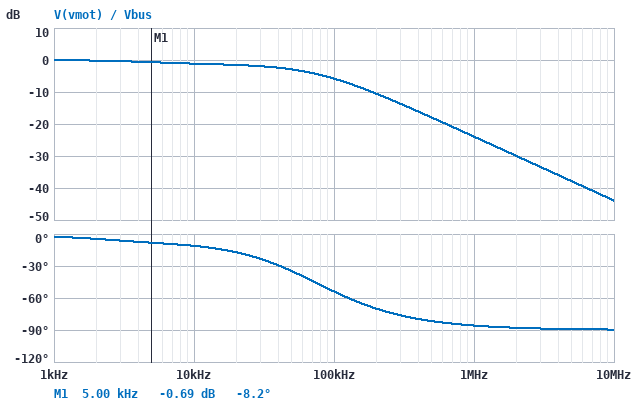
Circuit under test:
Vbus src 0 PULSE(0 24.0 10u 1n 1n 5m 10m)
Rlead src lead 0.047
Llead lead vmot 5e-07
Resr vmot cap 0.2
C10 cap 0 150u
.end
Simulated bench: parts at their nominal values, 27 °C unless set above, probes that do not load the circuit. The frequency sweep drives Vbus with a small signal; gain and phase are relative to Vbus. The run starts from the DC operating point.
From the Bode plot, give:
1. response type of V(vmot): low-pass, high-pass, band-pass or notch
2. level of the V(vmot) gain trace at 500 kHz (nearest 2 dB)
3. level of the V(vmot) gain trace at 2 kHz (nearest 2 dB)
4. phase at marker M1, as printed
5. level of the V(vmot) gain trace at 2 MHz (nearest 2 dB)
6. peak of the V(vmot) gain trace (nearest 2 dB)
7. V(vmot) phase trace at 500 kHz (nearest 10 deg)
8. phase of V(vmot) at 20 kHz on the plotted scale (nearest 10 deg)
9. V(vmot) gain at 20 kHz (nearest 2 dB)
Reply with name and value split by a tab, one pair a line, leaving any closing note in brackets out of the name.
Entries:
response type of V(vmot): low-pass, high-pass, band-pass or notch	low-pass
level of the V(vmot) gain trace at 500 kHz	-18 dB
level of the V(vmot) gain trace at 2 kHz	0 dB
phase at marker M1, as printed	-8.2 deg
level of the V(vmot) gain trace at 2 MHz	-30 dB
peak of the V(vmot) gain trace	0 dB
V(vmot) phase trace at 500 kHz	-80 deg
phase of V(vmot) at 20 kHz on the plotted scale	-20 deg
V(vmot) gain at 20 kHz	-2 dB
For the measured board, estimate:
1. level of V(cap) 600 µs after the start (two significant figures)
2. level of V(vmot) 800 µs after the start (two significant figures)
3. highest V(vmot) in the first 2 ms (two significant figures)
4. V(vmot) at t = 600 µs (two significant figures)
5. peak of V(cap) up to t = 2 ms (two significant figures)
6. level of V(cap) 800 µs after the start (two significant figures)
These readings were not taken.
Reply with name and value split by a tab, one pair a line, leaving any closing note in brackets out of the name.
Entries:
level of V(cap) 600 µs after the start	24 V
level of V(vmot) 800 µs after the start	24 V
highest V(vmot) in the first 2 ms	24 V
V(vmot) at t = 600 µs	24 V
peak of V(cap) up to t = 2 ms	24 V
level of V(cap) 800 µs after the start	24 V
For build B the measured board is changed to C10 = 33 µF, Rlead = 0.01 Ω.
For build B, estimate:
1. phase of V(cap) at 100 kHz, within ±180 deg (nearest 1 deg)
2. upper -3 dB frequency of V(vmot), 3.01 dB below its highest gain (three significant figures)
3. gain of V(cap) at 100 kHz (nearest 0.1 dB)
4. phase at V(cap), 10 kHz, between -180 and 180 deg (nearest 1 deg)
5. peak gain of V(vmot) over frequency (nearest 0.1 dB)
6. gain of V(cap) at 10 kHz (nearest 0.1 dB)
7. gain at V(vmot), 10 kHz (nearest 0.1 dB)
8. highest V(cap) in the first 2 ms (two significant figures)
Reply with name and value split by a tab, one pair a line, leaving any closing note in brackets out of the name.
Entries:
phase of V(cap) at 100 kHz, within ±180 deg	-142 deg
upper -3 dB frequency of V(vmot), 3.01 dB below its highest gain	69.2 kHz
gain of V(cap) at 100 kHz	-16.9 dB
phase at V(cap), 10 kHz, between -180 and 180 deg	-25 deg
peak gain of V(vmot) over frequency	1.3 dB
gain of V(cap) at 10 kHz	-0.3 dB
gain at V(vmot), 10 kHz	0.4 dB
highest V(cap) in the first 2 ms	24 V
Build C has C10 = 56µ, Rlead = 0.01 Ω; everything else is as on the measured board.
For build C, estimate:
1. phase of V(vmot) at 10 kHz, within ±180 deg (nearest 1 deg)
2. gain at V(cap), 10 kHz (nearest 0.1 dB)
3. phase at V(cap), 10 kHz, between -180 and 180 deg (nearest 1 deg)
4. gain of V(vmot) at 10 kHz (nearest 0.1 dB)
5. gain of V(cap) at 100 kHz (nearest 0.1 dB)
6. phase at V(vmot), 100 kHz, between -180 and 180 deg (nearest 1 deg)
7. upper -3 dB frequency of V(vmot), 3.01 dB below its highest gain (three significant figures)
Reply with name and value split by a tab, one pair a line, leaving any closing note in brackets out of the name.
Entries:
phase of V(vmot) at 10 kHz, within ±180 deg	-5 deg
gain at V(cap), 10 kHz	-1.3 dB
phase at V(cap), 10 kHz, between -180 and 180 deg	-40 deg
gain of V(vmot) at 10 kHz	0.5 dB
gain of V(cap) at 100 kHz	-21.9 dB
phase at V(vmot), 100 kHz, between -180 and 180 deg	-62 deg
upper -3 dB frequency of V(vmot), 3.01 dB below its highest gain	65.2 kHz
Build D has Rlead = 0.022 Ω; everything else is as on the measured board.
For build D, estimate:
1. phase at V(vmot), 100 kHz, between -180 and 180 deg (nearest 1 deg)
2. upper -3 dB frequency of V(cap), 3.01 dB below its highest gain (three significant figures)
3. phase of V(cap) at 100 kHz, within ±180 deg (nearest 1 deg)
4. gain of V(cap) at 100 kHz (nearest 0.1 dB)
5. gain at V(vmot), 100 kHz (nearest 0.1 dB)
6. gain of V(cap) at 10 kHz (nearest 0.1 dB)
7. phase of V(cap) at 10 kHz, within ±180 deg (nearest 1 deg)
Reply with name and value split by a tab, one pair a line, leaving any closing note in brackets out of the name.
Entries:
phase at V(vmot), 100 kHz, between -180 and 180 deg	-57 deg
upper -3 dB frequency of V(cap), 3.01 dB below its highest gain	5.12 kHz
phase of V(cap) at 100 kHz, within ±180 deg	-144 deg
gain of V(cap) at 100 kHz	-31.0 dB
gain at V(vmot), 100 kHz	-5.5 dB
gain of V(cap) at 10 kHz	-6.9 dB
phase of V(cap) at 10 kHz, within ±180 deg	-71 deg
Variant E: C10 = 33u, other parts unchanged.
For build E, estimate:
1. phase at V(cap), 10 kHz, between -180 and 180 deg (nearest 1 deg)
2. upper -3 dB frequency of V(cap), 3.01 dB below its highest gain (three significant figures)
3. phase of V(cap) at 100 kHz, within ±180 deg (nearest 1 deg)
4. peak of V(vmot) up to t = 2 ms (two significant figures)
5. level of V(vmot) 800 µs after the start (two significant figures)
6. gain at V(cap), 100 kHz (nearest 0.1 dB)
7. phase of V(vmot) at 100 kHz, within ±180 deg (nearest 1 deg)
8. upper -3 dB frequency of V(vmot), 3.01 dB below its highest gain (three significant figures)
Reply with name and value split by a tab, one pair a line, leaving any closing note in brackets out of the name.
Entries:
phase at V(cap), 10 kHz, between -180 and 180 deg	-29 deg
upper -3 dB frequency of V(cap), 3.01 dB below its highest gain	25.1 kHz
phase of V(cap) at 100 kHz, within ±180 deg	-137 deg
peak of V(vmot) up to t = 2 ms	25 V
level of V(vmot) 800 µs after the start	24 V
gain at V(cap), 100 kHz	-17.5 dB
phase of V(vmot) at 100 kHz, within ±180 deg	-61 deg
upper -3 dB frequency of V(vmot), 3.01 dB below its highest gain	70.5 kHz
